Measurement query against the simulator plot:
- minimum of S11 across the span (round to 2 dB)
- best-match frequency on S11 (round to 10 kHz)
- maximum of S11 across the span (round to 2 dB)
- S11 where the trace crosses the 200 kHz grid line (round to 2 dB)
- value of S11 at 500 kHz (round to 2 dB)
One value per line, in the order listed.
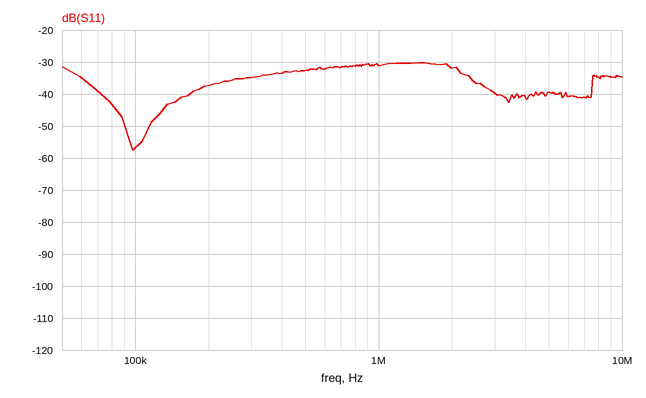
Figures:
-58 dB
100 kHz
-30 dB
-38 dB
-32 dB
